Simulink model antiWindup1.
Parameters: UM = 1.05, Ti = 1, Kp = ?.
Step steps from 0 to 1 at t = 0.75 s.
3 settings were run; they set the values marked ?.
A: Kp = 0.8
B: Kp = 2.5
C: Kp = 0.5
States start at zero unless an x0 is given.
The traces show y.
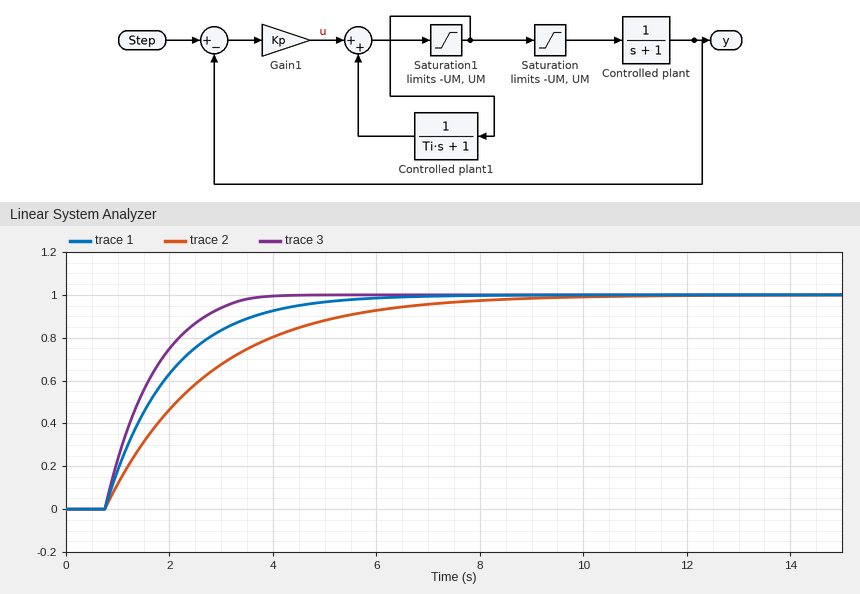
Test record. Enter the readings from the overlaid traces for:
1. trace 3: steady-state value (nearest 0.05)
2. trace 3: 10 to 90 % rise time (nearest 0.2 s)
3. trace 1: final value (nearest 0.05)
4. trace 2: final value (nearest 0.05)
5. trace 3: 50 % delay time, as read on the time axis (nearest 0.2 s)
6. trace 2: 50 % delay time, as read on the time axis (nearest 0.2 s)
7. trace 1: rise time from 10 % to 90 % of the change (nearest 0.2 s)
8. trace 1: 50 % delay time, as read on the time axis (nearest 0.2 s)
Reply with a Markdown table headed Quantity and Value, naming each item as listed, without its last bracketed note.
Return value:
| Quantity | Value |
|---|---|
| trace 3: steady-state value | 1.00 |
| trace 3: 10 to 90 % rise time | 1.8 s |
| trace 1: final value | 1.00 |
| trace 2: final value | 1.00 |
| trace 3: 50 % delay time, as read on the time axis | 1.4 s |
| trace 2: 50 % delay time, as read on the time axis | 2.2 s |
| trace 1: rise time from 10 % to 90 % of the change | 2.8 s |
| trace 1: 50 % delay time, as read on the time axis | 1.6 s |
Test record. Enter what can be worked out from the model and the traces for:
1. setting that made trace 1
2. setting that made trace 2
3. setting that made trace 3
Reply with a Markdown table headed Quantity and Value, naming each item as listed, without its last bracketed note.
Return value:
| Quantity | Value |
|---|---|
| setting that made trace 1 | A |
| setting that made trace 2 | C |
| setting that made trace 3 | B |
